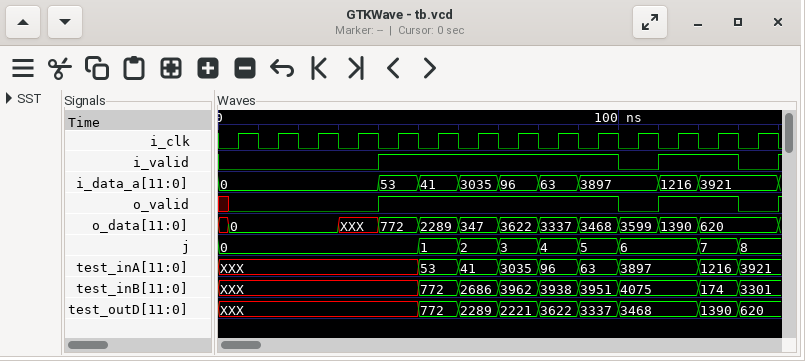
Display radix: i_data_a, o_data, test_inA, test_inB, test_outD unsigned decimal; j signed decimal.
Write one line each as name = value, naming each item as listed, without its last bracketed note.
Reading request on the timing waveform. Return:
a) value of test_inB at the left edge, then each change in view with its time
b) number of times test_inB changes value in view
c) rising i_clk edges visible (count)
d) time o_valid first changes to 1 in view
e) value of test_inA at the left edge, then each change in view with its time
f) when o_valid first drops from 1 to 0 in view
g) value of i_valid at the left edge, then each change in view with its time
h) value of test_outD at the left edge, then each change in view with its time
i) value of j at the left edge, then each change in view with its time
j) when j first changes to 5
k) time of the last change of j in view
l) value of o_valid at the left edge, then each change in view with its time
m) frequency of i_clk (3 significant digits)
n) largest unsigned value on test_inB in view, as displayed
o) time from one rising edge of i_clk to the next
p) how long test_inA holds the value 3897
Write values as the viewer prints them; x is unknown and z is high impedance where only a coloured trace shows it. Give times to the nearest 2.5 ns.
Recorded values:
value of test_inB at the left edge, then each change in view with its time = XXX, 772 at 50 ns, 2686 at 60 ns, 3962 at 70 ns, 3938 at 80 ns, 3951 at 90 ns, 4075 at 100 ns, 174 at 120 ns, 3301 at 130 ns
number of times test_inB changes value in view = 8
rising i_clk edges visible = 14
time o_valid first changes to 1 in view = 40 ns
value of test_inA at the left edge, then each change in view with its time = XXX, 53 at 50 ns, 41 at 60 ns, 3035 at 70 ns, 96 at 80 ns, 63 at 90 ns, 3897 at 100 ns, 1216 at 120 ns, 3921 at 130 ns
when o_valid first drops from 1 to 0 in view = 100 ns
value of i_valid at the left edge, then each change in view with its time = 0, 1 at 40 ns, 0 at 100 ns, 1 at 110 ns, 0 at 130 ns, 1 at 140 ns
value of test_outD at the left edge, then each change in view with its time = XXX, 772 at 50 ns, 2289 at 60 ns, 2221 at 70 ns, 3622 at 80 ns, 3337 at 90 ns, 3468 at 100 ns, 1390 at 120 ns, 620 at 130 ns
value of j at the left edge, then each change in view with its time = 0, 1 at 50 ns, 2 at 60 ns, 3 at 70 ns, 4 at 80 ns, 5 at 90 ns, 6 at 100 ns, 7 at 120 ns, 8 at 130 ns
when j first changes to 5 = 90 ns
time of the last change of j in view = 130 ns
value of o_valid at the left edge, then each change in view with its time = x, 0 at 2.5 ns, 1 at 40 ns, 0 at 100 ns, 1 at 110 ns, 0 at 130 ns, 1 at 140 ns
frequency of i_clk = 100 MHz
largest unsigned value on test_inB in view, as displayed = 4075
time from one rising edge of i_clk to the next = 10 ns
how long test_inA holds the value 3897 = 20 ns
